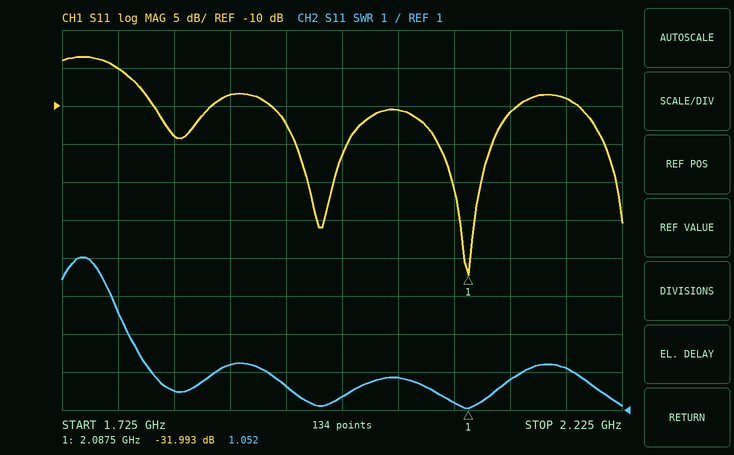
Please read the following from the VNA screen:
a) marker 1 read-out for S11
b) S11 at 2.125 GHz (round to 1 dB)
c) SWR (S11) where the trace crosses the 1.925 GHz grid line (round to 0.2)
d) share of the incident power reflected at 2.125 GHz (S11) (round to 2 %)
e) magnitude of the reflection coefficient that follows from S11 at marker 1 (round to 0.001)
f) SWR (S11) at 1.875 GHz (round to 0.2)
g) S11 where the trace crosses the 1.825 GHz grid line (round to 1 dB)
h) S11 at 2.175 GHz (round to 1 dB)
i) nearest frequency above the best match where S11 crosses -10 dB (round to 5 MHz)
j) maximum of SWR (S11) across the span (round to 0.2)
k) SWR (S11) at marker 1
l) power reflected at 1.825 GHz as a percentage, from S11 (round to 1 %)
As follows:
-31.993 dB
-11 dB
1.6
8 %
0.025
2.2
-14 dB
-9 dB
2.130 GHz
5.0
1.052
4 %
